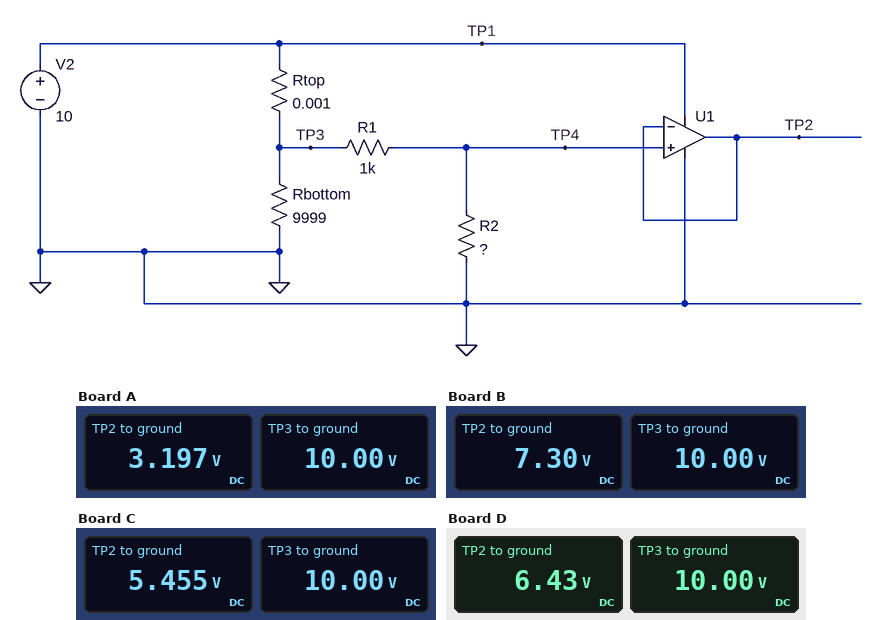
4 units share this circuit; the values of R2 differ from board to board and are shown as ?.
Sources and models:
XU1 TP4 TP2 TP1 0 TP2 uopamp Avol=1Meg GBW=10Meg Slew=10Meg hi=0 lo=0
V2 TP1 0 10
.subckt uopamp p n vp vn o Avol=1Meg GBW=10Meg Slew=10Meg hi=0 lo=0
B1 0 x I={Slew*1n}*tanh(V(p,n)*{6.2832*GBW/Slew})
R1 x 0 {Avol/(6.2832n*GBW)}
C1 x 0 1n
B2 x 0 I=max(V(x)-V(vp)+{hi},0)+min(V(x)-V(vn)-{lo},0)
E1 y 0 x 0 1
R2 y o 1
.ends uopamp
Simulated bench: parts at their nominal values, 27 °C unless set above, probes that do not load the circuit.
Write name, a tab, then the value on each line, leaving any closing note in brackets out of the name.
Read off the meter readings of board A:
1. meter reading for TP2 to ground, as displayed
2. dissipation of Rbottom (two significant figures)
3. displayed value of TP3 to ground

meter reading for TP2 to ground, as displayed	3.197 V
dissipation of Rbottom	10 mW
displayed value of TP3 to ground	10.00 V
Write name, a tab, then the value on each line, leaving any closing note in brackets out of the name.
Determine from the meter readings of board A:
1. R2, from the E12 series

R2, from the E12 series	470 Ω
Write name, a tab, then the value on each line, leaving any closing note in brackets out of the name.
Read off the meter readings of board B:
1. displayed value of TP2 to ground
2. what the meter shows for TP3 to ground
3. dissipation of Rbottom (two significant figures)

displayed value of TP2 to ground	7.30 V
what the meter shows for TP3 to ground	10.00 V
dissipation of Rbottom	10 mW
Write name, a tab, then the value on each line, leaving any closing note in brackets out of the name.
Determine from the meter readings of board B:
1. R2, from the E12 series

R2, from the E12 series	2.7 kΩ
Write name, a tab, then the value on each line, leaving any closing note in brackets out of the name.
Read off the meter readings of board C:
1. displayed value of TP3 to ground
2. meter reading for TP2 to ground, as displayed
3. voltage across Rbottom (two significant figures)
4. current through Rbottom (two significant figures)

displayed value of TP3 to ground	10.00 V
meter reading for TP2 to ground, as displayed	5.455 V
voltage across Rbottom	10 V
current through Rbottom	1.0 mA
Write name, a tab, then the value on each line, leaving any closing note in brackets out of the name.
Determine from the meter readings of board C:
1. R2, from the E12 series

R2, from the E12 series	1.2 kΩ
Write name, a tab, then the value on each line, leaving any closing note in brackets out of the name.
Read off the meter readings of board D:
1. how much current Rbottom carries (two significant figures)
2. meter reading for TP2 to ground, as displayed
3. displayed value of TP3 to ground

how much current Rbottom carries	1.0 mA
meter reading for TP2 to ground, as displayed	6.43 V
displayed value of TP3 to ground	10.00 V
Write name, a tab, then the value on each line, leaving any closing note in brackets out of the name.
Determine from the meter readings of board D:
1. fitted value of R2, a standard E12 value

fitted value of R2, a standard E12 value	1.8 kΩ
